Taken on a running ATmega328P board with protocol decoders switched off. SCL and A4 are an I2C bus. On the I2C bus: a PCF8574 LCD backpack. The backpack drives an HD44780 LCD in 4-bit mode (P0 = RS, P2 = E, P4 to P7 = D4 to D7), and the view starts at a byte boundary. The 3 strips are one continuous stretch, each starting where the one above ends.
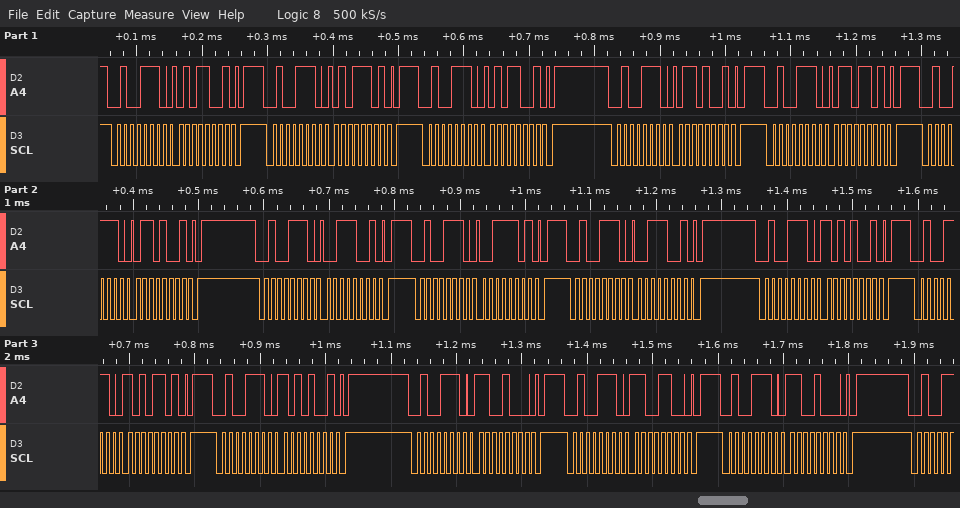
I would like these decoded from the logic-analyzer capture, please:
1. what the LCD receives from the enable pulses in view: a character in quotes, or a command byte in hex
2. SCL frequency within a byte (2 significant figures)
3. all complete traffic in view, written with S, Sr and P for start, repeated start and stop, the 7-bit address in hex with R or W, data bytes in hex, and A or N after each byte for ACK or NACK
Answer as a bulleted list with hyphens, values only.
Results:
- 'V' ':'
- 100 kHz
- S 27W A 59 A P S 27W A 5D A P S 27W A 59 A P S 27W A 69 A P S 27W A 6D A P S 27W A 69 A P S 27W A 39 A P S 27W A 3D A P S 27W A 39 A P S 27W A A9 A P S 27W A AD A P S 27W A A9 A P S 27W A C8 A P S 27W A CC A P S 27W A C8 A P
